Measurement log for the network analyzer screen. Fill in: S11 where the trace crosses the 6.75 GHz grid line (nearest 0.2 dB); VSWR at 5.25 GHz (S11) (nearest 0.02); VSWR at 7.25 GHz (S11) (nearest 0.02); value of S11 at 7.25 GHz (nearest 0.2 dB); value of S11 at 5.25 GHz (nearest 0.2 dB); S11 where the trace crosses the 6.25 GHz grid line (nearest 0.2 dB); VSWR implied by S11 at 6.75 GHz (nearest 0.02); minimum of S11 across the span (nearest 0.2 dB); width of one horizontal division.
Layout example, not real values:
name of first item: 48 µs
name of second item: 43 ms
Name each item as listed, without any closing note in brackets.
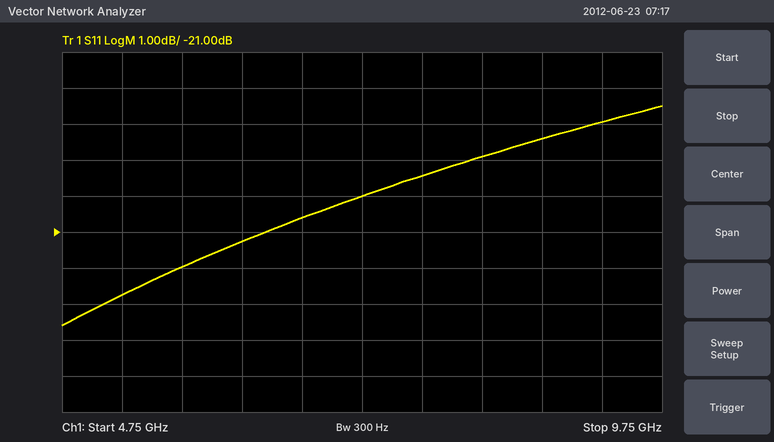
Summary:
S11 where the trace crosses the 6.75 GHz grid line: -20.6 dB
VSWR at 5.25 GHz (S11): 1.16
VSWR at 7.25 GHz (S11): 1.22
value of S11 at 7.25 GHz: -20.0 dB
value of S11 at 5.25 GHz: -22.8 dB
S11 where the trace crosses the 6.25 GHz grid line: -21.2 dB
VSWR implied by S11 at 6.75 GHz: 1.20
minimum of S11 across the span: -23.6 dB
width of one horizontal division: 500 MHz
